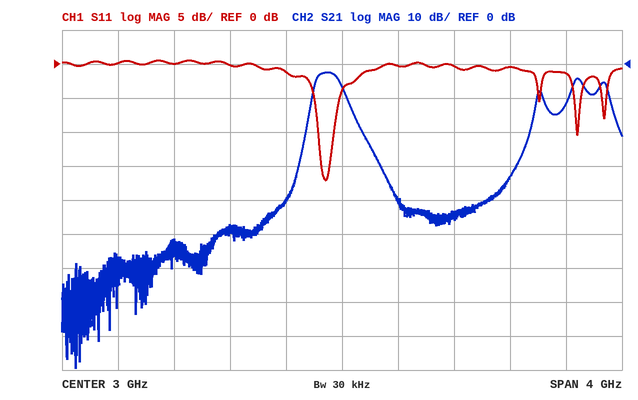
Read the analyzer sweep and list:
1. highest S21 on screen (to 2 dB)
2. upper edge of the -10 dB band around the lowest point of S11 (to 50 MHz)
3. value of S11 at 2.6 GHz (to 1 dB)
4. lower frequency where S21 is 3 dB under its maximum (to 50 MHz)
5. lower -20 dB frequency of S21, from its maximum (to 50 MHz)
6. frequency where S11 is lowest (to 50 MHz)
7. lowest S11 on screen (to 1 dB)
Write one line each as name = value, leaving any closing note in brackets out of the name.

highest S21 on screen = -2 dB
upper edge of the -10 dB band around the lowest point of S11 = 2.95 GHz
value of S11 at 2.6 GHz = -1 dB
lower frequency where S21 is 3 dB under its maximum = 2.80 GHz
lower -20 dB frequency of S21, from its maximum = 2.75 GHz
frequency where S11 is lowest = 2.90 GHz
lowest S11 on screen = -17 dB
